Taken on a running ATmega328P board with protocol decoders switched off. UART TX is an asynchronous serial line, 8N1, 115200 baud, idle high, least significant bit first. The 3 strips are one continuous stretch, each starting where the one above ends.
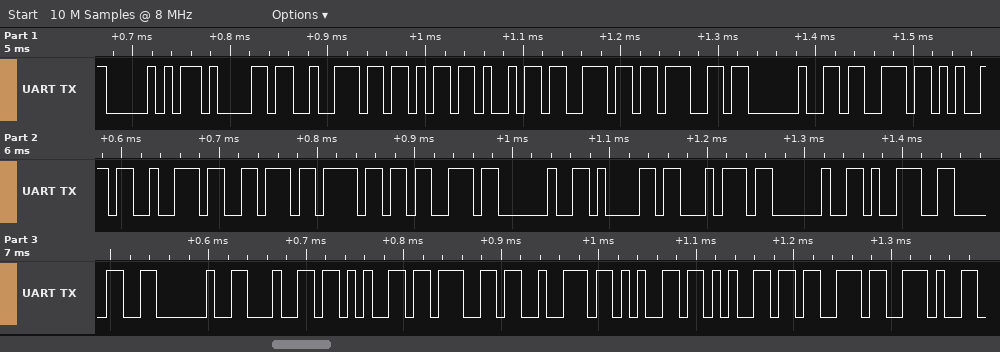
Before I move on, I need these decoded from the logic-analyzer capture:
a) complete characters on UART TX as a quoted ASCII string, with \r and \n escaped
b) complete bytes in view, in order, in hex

"Parking servos at 90 degrees."
50 61 72 6B 69 6E 67 20 73 65 72 76 6F 73 20 61 74 20 39 30 20 64 65 67 72 65 65 73 2E
